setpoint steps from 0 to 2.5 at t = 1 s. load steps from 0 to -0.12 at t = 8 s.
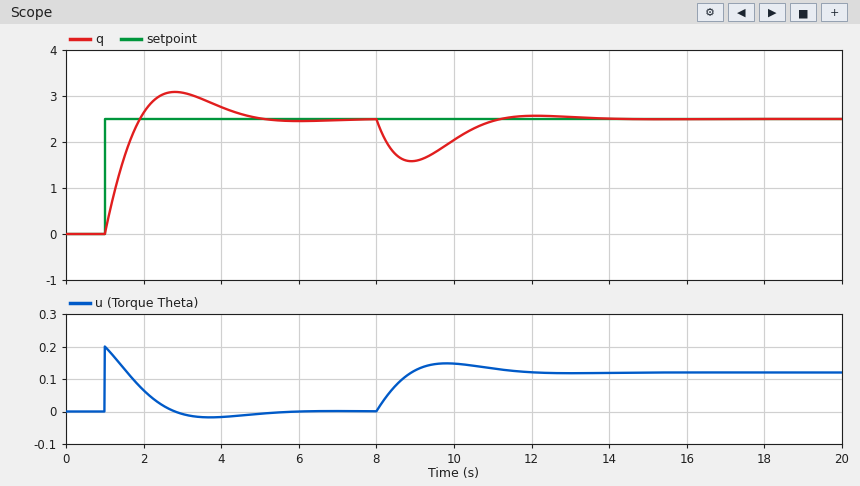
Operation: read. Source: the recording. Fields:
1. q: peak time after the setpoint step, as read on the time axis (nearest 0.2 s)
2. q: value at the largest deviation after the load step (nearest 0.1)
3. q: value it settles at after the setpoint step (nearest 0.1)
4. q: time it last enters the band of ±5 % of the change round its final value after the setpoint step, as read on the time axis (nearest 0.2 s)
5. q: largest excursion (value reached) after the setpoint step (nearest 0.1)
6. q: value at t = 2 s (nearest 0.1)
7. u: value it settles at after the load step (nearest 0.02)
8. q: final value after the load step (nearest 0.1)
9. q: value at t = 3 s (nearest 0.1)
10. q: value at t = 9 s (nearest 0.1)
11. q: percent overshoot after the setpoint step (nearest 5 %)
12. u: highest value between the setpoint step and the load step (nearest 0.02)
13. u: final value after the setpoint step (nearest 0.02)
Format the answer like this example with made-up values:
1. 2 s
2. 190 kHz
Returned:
1. 2.8 s
2. 1.6
3. 2.5
4. 4.4 s
5. 3.1
6. 2.6
7. 0.12
8. 2.5
9. 3.1
10. 1.6
11. 25 %
12. 0.20
13. 0.00
